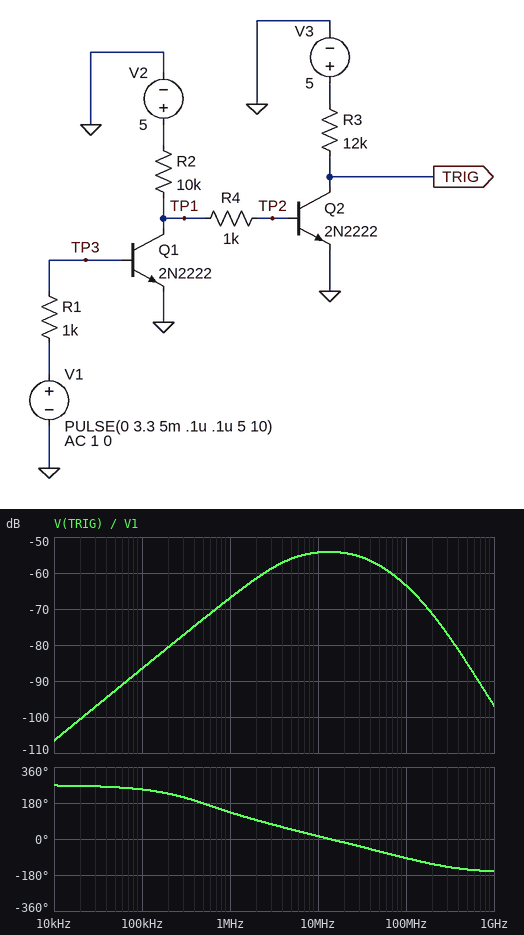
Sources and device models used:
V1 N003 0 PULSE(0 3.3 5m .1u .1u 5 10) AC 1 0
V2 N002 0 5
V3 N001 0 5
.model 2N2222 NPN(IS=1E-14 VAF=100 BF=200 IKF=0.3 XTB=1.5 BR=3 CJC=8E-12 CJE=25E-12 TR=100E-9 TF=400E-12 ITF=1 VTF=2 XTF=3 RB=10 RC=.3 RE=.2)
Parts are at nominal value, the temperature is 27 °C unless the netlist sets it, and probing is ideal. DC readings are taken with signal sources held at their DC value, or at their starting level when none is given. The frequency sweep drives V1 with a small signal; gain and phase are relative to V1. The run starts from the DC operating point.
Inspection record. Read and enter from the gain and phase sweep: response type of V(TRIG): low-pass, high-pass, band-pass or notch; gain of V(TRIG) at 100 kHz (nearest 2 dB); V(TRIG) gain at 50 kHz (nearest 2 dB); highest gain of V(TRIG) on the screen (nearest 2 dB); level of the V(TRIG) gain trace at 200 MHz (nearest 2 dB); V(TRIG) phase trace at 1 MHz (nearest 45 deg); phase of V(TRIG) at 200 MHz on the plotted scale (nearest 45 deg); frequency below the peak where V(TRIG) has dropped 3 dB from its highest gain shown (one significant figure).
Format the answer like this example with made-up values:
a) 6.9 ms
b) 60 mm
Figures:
a) band-pass
b) -86 dB
c) -92 dB
d) -54 dB
e) -72 dB
f) 135 deg
g) -135 deg
h) 4 MHz
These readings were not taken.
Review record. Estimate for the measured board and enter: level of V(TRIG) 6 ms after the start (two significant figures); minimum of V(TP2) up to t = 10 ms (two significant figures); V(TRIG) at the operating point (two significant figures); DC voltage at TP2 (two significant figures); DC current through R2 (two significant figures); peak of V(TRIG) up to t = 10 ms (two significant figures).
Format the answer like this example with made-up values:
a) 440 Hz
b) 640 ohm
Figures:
a) 5.0 V
b) 9.8 mV
c) 14 mV
d) 680 mV
e) 390 µA
f) 5.0 V
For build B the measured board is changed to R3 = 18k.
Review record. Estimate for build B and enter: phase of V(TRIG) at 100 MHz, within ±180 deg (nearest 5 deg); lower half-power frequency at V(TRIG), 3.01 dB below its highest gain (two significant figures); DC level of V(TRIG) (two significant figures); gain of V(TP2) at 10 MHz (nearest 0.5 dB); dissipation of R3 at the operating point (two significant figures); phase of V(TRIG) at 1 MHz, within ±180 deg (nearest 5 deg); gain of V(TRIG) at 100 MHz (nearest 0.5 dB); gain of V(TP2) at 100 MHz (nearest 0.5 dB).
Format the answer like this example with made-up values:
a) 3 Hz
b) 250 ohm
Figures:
a) -95 deg
b) 4.0 MHz
c) 12 mV
d) -49.0 dB
e) 1.4 mW
f) 125 deg
g) -63.0 dB
h) -58.0 dB
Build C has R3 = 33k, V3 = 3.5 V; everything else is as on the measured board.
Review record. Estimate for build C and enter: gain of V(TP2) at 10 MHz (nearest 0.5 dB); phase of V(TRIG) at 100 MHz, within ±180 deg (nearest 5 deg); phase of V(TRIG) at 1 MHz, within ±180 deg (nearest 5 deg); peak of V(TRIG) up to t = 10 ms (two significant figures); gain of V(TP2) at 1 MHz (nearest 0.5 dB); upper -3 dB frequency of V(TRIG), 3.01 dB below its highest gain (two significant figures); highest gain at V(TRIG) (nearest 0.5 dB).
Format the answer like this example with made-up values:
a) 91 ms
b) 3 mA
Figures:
a) -48.5 dB
b) -100 deg
c) 110 deg
d) 3.5 V
e) -57.5 dB
f) 43 MHz
g) -52.5 dB
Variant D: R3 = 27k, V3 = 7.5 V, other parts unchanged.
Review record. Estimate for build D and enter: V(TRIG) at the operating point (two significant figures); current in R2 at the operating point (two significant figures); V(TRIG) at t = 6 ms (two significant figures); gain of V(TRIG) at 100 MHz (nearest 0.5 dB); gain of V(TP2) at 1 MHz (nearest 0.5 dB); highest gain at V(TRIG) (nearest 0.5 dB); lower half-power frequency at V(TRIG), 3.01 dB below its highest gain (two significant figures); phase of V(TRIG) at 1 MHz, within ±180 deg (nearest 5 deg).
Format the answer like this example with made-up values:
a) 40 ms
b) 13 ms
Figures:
a) 12 mV
b) 390 µA
c) 7.5 V
d) -63.0 dB
e) -58.0 dB
f) -53.5 dB
g) 4.0 MHz
h) 125 deg
